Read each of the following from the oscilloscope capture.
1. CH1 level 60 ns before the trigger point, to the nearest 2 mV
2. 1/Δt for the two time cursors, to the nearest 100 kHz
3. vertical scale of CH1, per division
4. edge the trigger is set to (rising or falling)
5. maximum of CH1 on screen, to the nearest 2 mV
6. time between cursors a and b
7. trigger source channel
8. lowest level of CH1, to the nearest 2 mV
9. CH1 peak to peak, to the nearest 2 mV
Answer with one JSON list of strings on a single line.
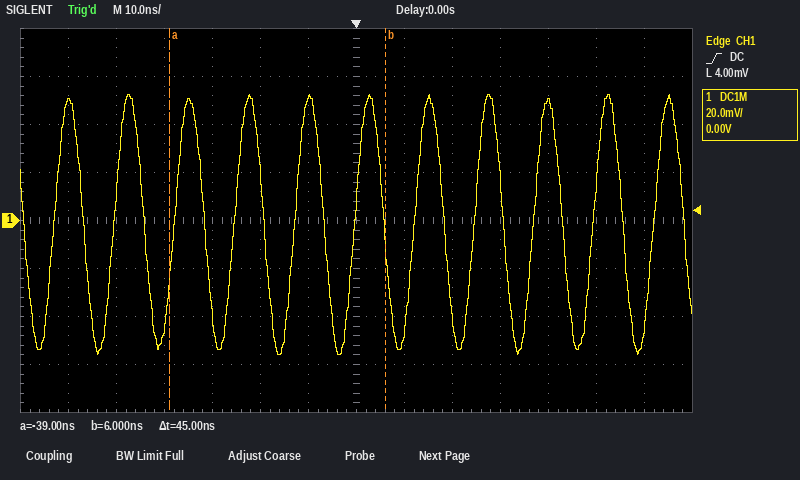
["50 mV", "22.2 MHz", "20 mV", "rising", "52 mV", "45 ns", "CH1", "-56 mV", "108 mV"]
